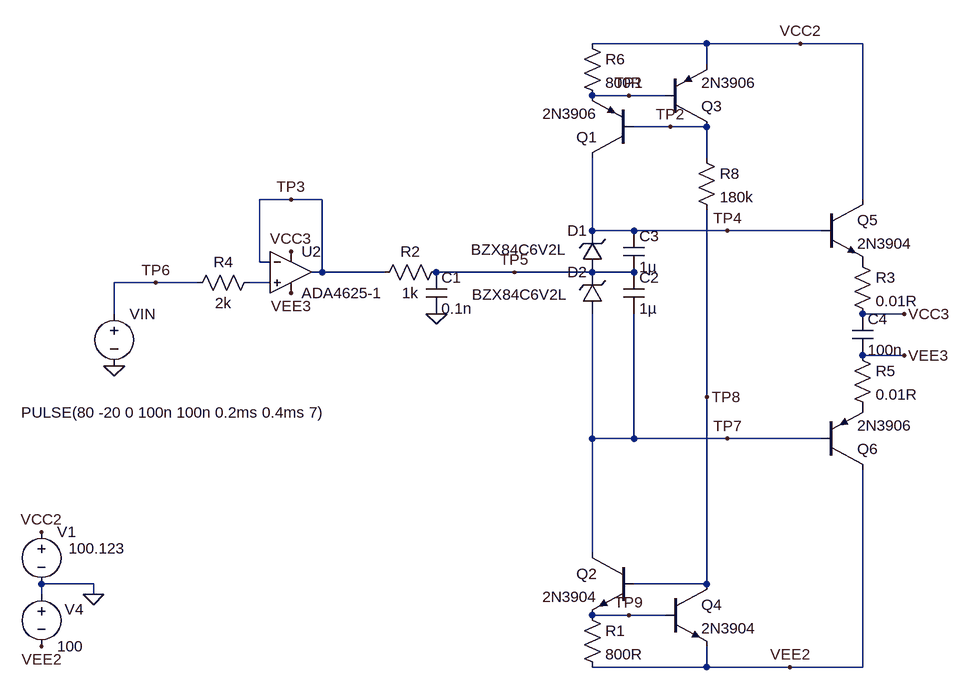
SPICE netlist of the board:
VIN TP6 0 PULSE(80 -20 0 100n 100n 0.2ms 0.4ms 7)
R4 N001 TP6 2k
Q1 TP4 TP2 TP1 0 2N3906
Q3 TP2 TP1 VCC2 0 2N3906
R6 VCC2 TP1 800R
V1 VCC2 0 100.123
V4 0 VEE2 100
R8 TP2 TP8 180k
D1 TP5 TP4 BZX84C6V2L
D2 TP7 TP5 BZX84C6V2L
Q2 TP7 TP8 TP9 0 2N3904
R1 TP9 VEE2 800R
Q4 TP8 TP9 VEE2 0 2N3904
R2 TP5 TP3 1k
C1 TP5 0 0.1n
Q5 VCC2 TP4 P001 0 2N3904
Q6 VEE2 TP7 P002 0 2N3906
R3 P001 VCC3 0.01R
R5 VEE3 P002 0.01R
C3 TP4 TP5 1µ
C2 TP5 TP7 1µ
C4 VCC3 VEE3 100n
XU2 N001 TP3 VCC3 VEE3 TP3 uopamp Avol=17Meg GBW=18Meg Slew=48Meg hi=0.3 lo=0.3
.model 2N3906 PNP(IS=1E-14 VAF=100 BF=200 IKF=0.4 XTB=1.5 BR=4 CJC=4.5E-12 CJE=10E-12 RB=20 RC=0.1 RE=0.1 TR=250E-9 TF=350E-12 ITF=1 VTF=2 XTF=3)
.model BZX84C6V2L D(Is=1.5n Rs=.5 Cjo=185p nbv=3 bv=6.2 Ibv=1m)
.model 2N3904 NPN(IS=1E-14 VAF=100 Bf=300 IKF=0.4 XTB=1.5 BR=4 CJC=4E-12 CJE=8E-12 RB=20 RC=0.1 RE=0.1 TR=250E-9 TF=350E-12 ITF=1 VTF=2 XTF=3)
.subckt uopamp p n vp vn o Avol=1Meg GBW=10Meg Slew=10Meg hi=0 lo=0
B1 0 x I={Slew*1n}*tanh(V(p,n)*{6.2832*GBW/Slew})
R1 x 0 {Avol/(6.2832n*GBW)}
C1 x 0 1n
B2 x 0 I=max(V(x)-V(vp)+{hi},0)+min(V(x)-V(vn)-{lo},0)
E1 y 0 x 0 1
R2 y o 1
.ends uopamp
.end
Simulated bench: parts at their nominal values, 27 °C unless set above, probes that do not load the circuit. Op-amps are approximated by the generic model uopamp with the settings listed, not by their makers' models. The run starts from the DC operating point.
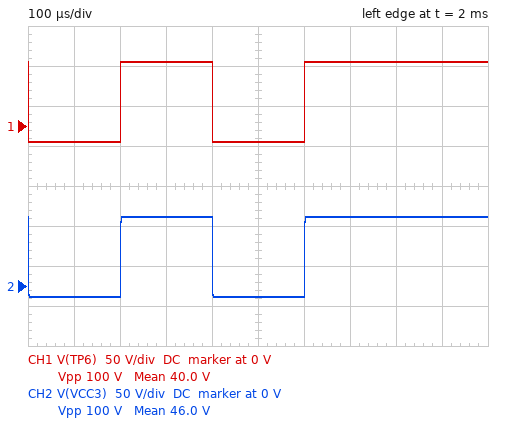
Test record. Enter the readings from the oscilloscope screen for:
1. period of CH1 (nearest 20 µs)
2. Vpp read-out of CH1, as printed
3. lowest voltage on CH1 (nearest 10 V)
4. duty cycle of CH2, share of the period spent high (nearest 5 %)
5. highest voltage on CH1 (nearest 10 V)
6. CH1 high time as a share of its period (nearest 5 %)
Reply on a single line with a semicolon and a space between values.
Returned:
400 µs; 100 V; -20 V; 50 %; 80 V; 50 %
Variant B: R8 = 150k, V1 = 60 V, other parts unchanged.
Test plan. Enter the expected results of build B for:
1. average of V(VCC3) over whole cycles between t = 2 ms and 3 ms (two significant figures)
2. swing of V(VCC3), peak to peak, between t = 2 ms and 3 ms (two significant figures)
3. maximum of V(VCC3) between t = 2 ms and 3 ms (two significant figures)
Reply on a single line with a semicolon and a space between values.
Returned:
20 V; 78 V; 59 V
